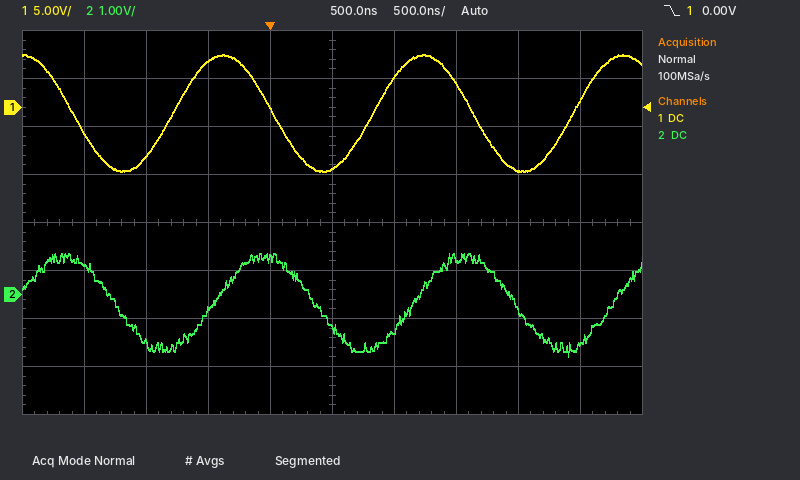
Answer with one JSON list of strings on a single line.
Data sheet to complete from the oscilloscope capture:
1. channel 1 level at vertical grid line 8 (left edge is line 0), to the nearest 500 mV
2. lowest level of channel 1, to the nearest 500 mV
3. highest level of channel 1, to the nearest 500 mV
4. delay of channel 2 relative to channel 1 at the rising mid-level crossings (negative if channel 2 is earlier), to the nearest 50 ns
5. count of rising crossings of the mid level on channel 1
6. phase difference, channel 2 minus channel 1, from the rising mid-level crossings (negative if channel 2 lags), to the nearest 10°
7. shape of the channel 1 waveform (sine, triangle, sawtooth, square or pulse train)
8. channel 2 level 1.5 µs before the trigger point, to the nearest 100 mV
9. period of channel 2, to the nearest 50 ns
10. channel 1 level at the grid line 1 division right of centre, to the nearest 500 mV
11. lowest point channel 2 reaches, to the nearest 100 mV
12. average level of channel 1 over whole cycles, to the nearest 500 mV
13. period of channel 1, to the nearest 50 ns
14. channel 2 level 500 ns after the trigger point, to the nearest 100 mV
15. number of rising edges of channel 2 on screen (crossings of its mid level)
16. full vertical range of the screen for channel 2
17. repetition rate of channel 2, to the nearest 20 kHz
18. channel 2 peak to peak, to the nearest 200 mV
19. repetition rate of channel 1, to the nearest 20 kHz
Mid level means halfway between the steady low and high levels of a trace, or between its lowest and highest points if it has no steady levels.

["-6.5 V", "-6.5 V", "5.5 V", "+300 ns", "3", "-70°", "sine", "600 mV", "1.60 µs", "3.0 V", "-1.3 V", "-500 mV", "1.60 µs", "-700 mV", "3", "8 V", "620 kHz", "2.2 V", "620 kHz"]
